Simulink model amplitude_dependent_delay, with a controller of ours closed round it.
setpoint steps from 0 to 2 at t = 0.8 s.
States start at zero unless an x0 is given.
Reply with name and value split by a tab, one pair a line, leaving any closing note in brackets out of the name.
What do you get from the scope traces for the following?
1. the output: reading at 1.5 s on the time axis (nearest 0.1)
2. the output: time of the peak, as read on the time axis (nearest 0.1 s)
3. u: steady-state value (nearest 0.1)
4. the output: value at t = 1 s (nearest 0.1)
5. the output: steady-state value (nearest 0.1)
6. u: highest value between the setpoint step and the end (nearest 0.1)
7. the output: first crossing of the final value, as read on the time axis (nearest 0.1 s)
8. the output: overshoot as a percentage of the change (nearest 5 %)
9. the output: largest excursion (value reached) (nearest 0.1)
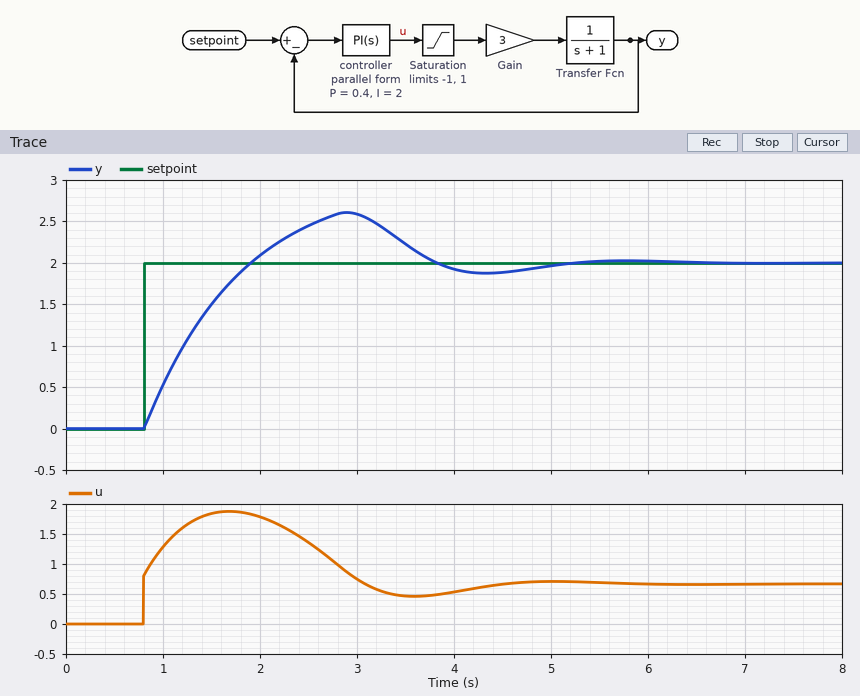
the output: reading at 1.5 s on the time axis	1.5
the output: time of the peak, as read on the time axis	2.9 s
u: steady-state value	0.7
the output: value at t = 1 s	0.5
the output: steady-state value	2.0
u: highest value between the setpoint step and the end	1.9
the output: first crossing of the final value, as read on the time axis	1.9 s
the output: overshoot as a percentage of the change	30 %
the output: largest excursion (value reached)	2.6
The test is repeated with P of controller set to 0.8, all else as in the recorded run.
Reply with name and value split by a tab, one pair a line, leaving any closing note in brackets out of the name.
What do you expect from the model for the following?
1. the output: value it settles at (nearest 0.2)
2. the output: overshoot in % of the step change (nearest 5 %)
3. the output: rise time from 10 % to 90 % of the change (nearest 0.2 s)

the output: value it settles at	2.0
the output: overshoot in % of the step change	25 %
the output: rise time from 10 % to 90 % of the change	0.8 s
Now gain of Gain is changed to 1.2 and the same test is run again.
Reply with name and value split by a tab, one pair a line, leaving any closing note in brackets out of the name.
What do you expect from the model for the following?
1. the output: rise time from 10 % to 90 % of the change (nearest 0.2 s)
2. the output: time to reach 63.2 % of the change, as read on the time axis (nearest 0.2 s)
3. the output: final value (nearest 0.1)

the output: rise time from 10 % to 90 % of the change	2.2 s
the output: time to reach 63.2 % of the change, as read on the time axis	1.8 s
the output: final value	1.2
